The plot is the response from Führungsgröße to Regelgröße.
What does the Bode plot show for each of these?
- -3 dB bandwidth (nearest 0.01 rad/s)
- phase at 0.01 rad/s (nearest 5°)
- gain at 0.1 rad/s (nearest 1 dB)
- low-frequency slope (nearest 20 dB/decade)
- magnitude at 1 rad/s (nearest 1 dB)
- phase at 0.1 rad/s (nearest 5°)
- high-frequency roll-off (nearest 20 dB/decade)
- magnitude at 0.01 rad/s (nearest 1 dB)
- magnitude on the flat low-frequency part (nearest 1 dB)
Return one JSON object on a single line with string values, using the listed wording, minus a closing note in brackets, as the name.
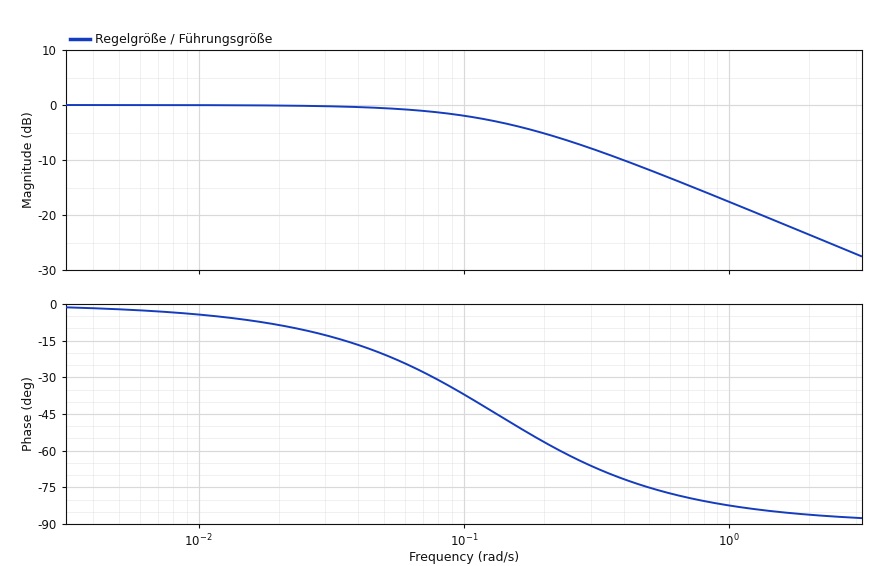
{"-3 dB bandwidth": "0.13 rad/s", "phase at 0.01 rad/s": "-5°", "gain at 0.1 rad/s": "-2 dB", "low-frequency slope": "0 dB/decade", "magnitude at 1 rad/s": "-18 dB", "phase at 0.1 rad/s": "-35°", "high-frequency roll-off": "-20 dB/decade", "magnitude at 0.01 rad/s": "0 dB", "magnitude on the flat low-frequency part": "0 dB"}
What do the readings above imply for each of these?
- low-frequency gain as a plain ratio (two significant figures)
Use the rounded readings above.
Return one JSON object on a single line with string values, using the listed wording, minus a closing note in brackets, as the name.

{"low-frequency gain as a plain ratio": "1.0"}
